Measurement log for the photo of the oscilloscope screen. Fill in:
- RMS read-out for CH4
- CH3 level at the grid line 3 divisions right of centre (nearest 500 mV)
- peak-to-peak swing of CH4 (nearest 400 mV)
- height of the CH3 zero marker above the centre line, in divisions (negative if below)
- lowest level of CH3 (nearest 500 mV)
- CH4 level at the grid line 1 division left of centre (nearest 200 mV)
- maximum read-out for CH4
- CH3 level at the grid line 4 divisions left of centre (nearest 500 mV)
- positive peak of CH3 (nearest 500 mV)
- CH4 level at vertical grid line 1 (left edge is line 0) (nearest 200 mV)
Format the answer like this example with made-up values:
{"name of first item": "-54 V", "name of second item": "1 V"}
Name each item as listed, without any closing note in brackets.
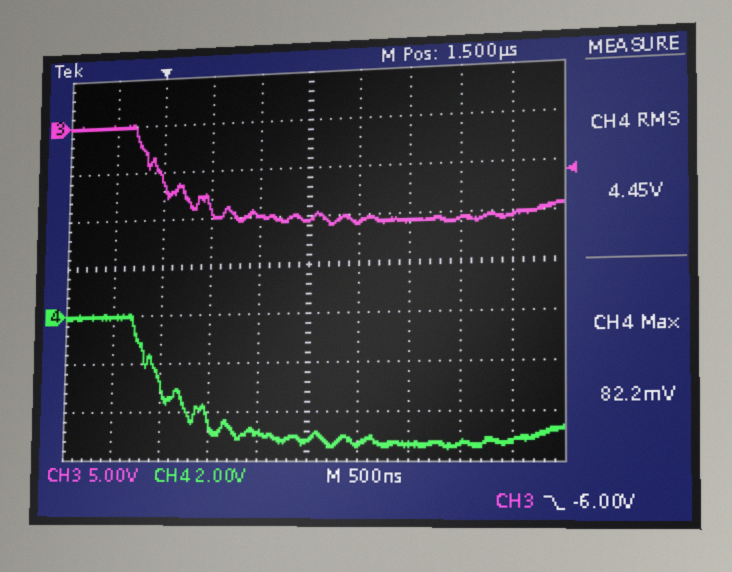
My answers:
{"RMS read-out for CH4": "4.45 V", "CH3 level at the grid line 3 divisions right of centre": "-10.5 V", "peak-to-peak swing of CH4": "5.6 V", "height of the CH3 zero marker above the centre line, in divisions": "+3.0 div", "lowest level of CH3": "-11.0 V", "CH4 level at the grid line 1 division left of centre": "-4.8 V", "maximum read-out for CH4": "82.2 mV", "CH3 level at the grid line 4 divisions left of centre": "0.0 V", "positive peak of CH3": "0.0 V", "CH4 level at vertical grid line 1 (left edge is line 0)": "0.0 V"}
